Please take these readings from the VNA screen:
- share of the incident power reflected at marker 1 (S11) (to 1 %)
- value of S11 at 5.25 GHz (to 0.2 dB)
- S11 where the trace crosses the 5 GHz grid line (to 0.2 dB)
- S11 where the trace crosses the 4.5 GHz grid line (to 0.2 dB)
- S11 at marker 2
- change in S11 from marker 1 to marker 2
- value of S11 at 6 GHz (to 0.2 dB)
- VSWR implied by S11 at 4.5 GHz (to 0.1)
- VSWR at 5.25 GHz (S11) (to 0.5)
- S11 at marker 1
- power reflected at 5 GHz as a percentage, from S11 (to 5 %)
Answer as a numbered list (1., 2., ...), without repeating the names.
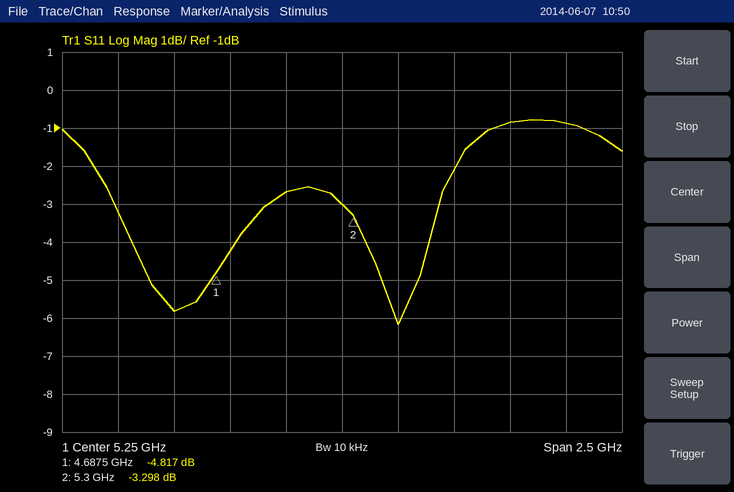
1. 33 %
2. -3.0 dB
3. -2.6 dB
4. -5.8 dB
5. -3.298 dB
6. 1.519 dB
7. -0.8 dB
8. 3.1
9. 6.0
10. -4.817 dB
11. 55 %
